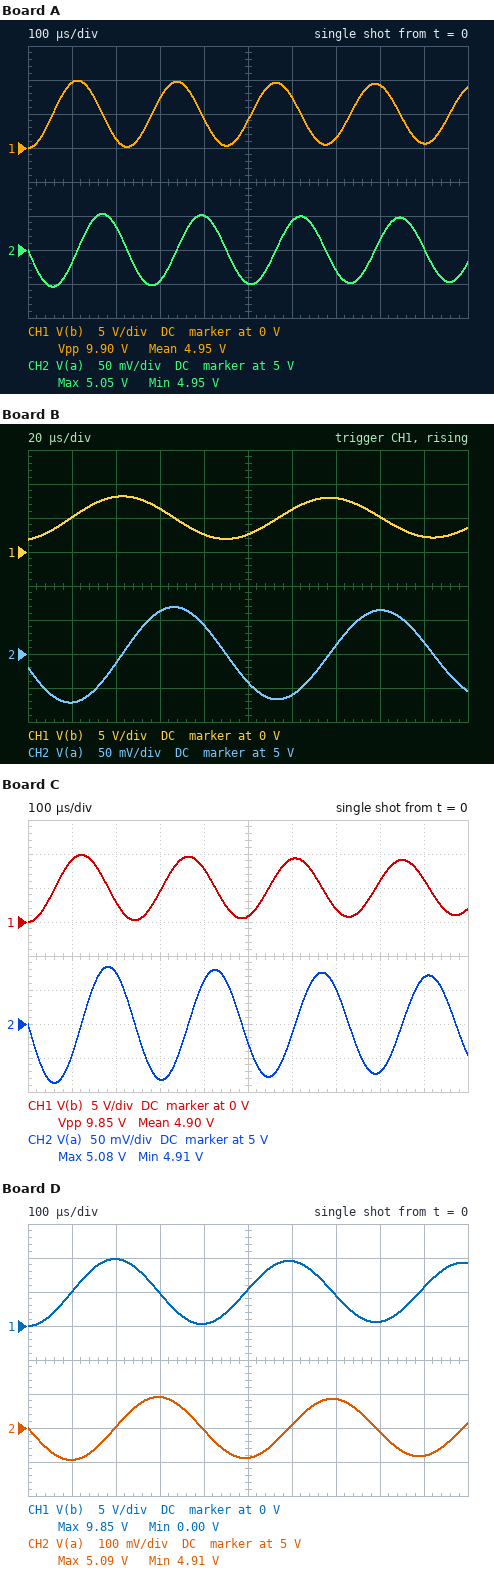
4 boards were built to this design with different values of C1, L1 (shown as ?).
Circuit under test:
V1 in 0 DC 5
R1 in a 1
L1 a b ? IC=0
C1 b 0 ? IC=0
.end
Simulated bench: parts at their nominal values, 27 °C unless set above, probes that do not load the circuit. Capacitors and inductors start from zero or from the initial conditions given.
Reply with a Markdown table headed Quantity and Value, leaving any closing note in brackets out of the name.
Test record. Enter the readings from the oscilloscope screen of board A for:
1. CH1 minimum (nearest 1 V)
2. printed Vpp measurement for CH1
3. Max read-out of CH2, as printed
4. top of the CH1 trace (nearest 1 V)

| Quantity | Value |
|---|---|
| CH1 minimum | 0 V |
| printed Vpp measurement for CH1 | 9.90 V |
| Max read-out of CH2, as printed | 5.05 V |
| top of the CH1 trace | 10 V |
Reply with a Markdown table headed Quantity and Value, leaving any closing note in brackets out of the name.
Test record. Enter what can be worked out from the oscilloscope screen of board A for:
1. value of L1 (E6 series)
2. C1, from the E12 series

| Quantity | Value |
|---|---|
| value of L1 | 3.3 mH |
| C1, from the E12 series | 390 nF |
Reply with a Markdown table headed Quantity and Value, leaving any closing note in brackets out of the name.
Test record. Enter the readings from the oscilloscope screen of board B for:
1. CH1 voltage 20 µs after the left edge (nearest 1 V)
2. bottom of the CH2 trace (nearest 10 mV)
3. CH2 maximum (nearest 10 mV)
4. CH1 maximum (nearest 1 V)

| Quantity | Value |
|---|---|
| CH1 voltage 20 µs after the left edge | 5 V |
| bottom of the CH2 trace | 4.93 V |
| CH2 maximum | 5.07 V |
| CH1 maximum | 8 V |
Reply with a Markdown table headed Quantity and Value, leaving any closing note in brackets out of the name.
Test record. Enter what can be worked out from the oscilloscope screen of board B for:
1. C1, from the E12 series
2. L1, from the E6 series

| Quantity | Value |
|---|---|
| C1, from the E12 series | 330 nF |
| L1, from the E6 series | 680 µH |
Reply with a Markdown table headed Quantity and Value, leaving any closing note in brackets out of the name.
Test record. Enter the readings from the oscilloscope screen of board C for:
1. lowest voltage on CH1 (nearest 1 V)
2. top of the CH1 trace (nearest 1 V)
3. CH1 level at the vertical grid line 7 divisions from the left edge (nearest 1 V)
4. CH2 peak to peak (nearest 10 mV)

| Quantity | Value |
|---|---|
| lowest voltage on CH1 | 0 V |
| top of the CH1 trace | 10 V |
| CH1 level at the vertical grid line 7 divisions from the left edge | 2 V |
| CH2 peak to peak | 170 mV |
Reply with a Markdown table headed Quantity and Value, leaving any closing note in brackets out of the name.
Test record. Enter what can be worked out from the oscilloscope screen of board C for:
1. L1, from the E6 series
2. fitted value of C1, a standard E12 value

| Quantity | Value |
|---|---|
| L1, from the E6 series | 2.2 mH |
| fitted value of C1, a standard E12 value | 680 nF |
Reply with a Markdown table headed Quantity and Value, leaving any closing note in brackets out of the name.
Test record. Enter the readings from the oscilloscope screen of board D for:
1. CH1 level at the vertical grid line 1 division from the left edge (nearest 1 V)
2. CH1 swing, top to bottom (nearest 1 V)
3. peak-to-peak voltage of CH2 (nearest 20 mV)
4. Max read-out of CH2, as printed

| Quantity | Value |
|---|---|
| CH1 level at the vertical grid line 1 division from the left edge | 5 V |
| CH1 swing, top to bottom | 10 V |
| peak-to-peak voltage of CH2 | 180 mV |
| Max read-out of CH2, as printed | 5.09 V |
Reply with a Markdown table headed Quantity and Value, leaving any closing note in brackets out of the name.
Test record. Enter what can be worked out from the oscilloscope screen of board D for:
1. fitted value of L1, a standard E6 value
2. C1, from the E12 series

| Quantity | Value |
|---|---|
| fitted value of L1, a standard E6 value | 3.3 mH |
| C1, from the E12 series | 1.2 µF |
